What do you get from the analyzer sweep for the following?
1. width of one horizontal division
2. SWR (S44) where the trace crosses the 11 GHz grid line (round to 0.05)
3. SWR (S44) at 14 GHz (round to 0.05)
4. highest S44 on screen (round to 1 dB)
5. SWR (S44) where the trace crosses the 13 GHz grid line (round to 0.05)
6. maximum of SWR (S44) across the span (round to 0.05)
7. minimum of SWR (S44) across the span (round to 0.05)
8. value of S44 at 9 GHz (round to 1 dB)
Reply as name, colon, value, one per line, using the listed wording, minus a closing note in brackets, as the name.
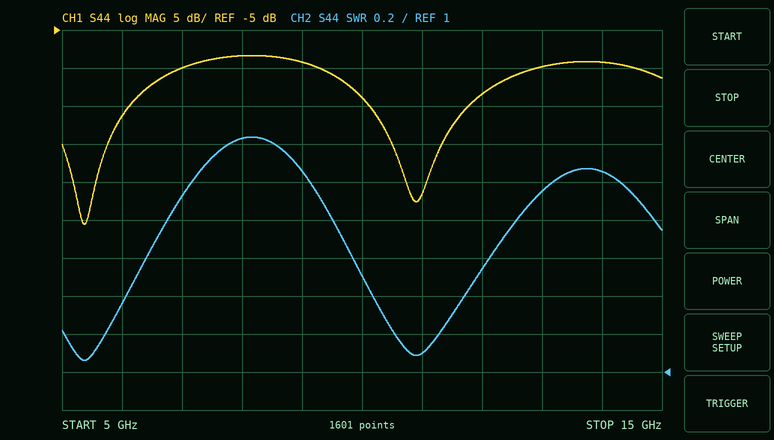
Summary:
width of one horizontal division: 1 GHz
SWR (S44) where the trace crosses the 11 GHz grid line: 1.10
SWR (S44) at 14 GHz: 2.05
highest S44 on screen: -8 dB
SWR (S44) where the trace crosses the 13 GHz grid line: 1.95
maximum of SWR (S44) across the span: 2.25
minimum of SWR (S44) across the span: 1.05
value of S44 at 9 GHz: -9 dB
